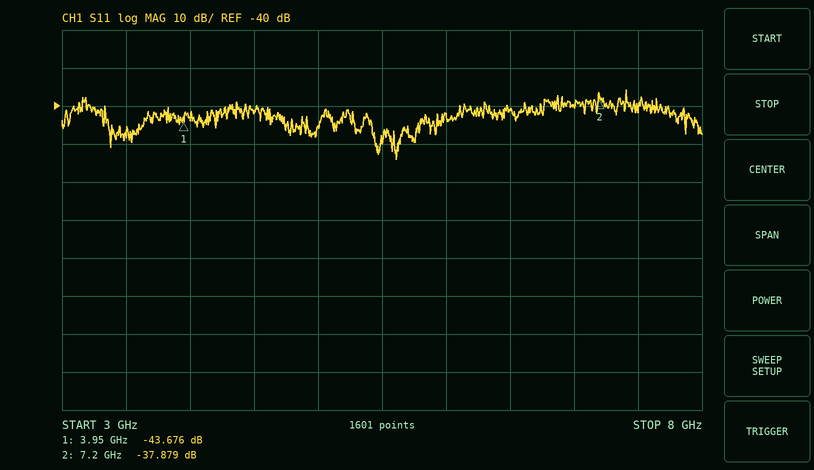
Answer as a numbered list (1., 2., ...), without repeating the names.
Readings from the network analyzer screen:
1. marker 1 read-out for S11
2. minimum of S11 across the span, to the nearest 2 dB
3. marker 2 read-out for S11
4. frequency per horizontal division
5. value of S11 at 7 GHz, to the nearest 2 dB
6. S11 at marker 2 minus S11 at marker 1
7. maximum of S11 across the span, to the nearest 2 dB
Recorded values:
1. -43.676 dB
2. -54 dB
3. -37.879 dB
4. 500 MHz
5. -40 dB
6. 5.797 dB
7. -36 dB
